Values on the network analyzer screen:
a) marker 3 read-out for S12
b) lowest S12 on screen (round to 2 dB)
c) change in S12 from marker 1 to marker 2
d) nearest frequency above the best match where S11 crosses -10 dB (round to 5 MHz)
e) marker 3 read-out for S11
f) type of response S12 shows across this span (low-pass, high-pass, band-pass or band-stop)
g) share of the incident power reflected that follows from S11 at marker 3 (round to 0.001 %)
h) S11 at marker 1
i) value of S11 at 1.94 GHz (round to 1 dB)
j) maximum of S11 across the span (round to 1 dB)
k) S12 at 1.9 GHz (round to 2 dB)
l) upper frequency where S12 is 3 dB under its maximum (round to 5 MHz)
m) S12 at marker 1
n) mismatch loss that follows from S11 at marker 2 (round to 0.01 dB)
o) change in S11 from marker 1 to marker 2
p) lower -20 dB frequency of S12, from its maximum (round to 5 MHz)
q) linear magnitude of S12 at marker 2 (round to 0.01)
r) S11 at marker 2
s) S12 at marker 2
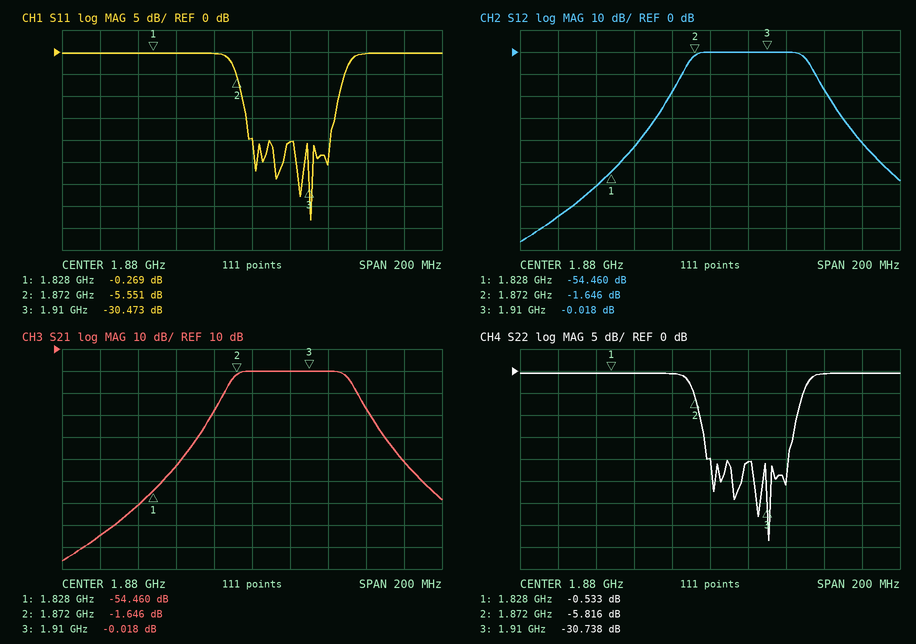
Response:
-0.018 dB
-86 dB
52.814 dB
1.925 GHz
-30.473 dB
band-pass
0.090 %
-0.269 dB
0 dB
0 dB
0 dB
1.930 GHz
-54.460 dB
1.42 dB
-5.282 dB
1.860 GHz
0.83
-5.551 dB
-1.646 dB
